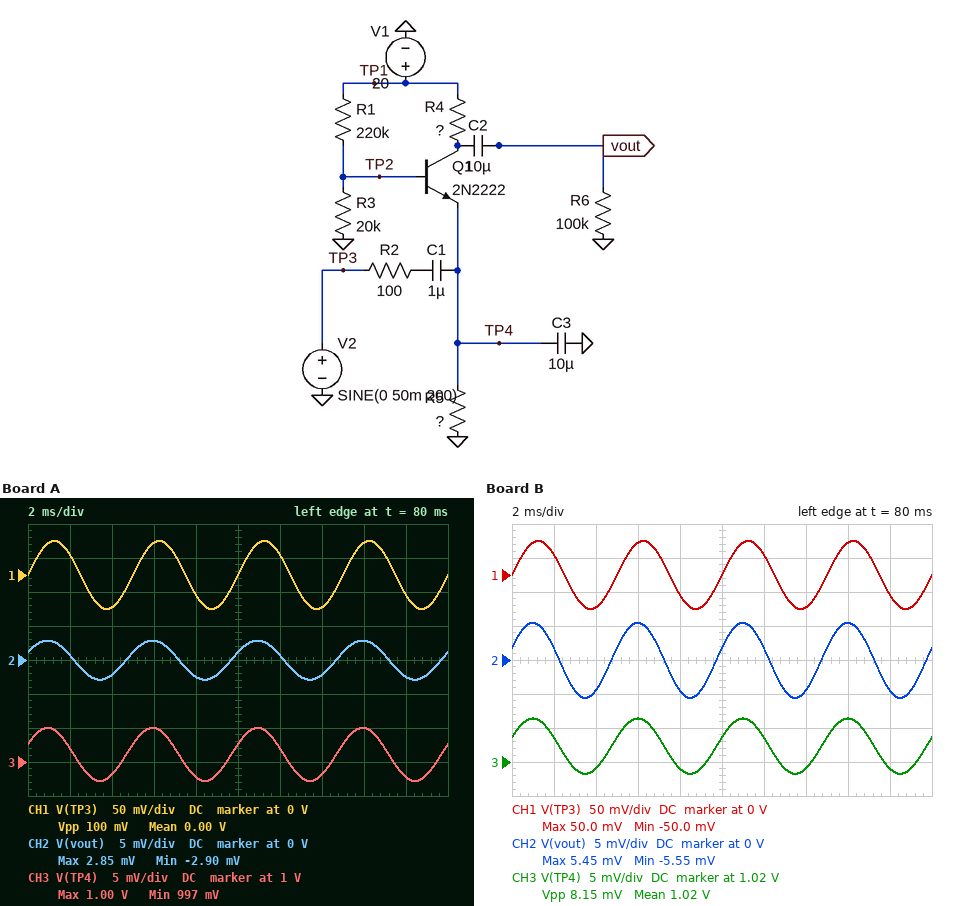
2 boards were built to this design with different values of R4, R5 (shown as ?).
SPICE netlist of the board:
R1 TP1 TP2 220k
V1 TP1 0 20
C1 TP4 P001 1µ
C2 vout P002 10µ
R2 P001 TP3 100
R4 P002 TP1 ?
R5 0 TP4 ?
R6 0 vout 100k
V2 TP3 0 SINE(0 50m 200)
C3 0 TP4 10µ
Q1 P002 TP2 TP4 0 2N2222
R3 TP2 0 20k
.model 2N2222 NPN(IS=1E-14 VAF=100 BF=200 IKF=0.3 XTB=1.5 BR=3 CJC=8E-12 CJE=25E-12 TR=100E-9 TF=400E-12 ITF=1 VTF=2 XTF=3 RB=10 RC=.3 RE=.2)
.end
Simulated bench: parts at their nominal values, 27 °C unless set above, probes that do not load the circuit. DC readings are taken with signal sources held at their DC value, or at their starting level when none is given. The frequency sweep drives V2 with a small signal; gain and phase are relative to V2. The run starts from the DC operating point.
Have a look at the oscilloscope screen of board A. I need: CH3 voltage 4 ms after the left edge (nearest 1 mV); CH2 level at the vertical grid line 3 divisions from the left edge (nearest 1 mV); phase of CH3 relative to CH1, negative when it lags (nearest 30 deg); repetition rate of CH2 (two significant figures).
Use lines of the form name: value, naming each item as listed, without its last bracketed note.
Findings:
CH3 voltage 4 ms after the left edge: 998 mV
CH2 level at the vertical grid line 3 divisions from the left edge: 3 mV
phase of CH3 relative to CH1, negative when it lags: 30 deg
repetition rate of CH2: 200 Hz
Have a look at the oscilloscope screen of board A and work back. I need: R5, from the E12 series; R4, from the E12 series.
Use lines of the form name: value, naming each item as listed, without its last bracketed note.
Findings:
R5, from the E12 series: 2.2 kΩ
R4, from the E12 series: 100 Ω
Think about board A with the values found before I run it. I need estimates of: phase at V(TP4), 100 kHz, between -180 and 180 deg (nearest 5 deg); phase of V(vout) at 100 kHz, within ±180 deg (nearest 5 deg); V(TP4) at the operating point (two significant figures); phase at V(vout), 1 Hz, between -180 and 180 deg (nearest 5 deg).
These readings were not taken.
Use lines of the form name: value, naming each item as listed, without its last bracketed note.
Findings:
phase at V(TP4), 100 kHz, between -180 and 180 deg: -90 deg
phase of V(vout) at 100 kHz, within ±180 deg: -100 deg
V(TP4) at the operating point: 1.0 V
phase at V(vout), 1 Hz, between -180 and 180 deg: 100 deg
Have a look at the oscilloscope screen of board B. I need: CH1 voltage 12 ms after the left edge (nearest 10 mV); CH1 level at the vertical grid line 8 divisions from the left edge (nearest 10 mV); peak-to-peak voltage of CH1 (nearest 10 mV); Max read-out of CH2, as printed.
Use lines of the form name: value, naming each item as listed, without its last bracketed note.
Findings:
CH1 voltage 12 ms after the left edge: 30 mV
CH1 level at the vertical grid line 8 divisions from the left edge: 50 mV
peak-to-peak voltage of CH1: 100 mV
Max read-out of CH2, as printed: 5.45 mV
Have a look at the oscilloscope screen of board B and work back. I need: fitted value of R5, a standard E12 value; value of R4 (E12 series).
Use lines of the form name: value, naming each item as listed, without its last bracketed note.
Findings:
fitted value of R5, a standard E12 value: 3.3 kΩ
value of R4: 220 Ω
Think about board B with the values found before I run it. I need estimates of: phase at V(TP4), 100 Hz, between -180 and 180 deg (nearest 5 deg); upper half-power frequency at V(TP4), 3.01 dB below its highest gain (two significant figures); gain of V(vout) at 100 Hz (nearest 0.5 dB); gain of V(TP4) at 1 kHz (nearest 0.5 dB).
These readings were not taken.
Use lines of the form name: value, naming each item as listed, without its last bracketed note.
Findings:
phase at V(TP4), 100 Hz, between -180 and 180 deg: 40 deg
upper half-power frequency at V(TP4), 3.01 dB below its highest gain: 1.9 kHz
gain of V(vout) at 100 Hz: -21.0 dB
gain of V(TP4) at 1 kHz: -22.0 dB
